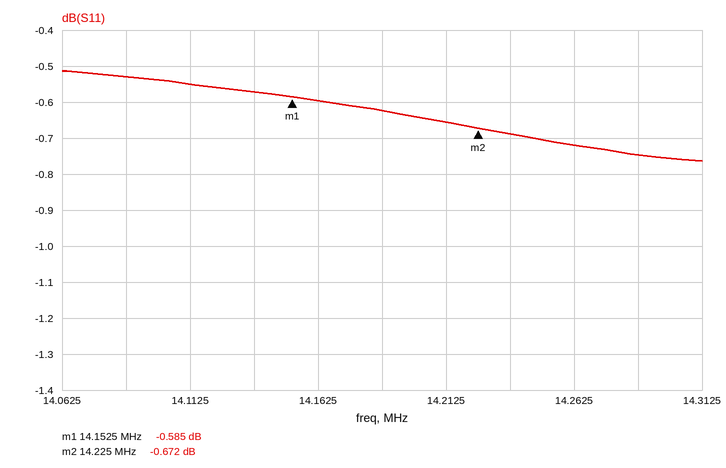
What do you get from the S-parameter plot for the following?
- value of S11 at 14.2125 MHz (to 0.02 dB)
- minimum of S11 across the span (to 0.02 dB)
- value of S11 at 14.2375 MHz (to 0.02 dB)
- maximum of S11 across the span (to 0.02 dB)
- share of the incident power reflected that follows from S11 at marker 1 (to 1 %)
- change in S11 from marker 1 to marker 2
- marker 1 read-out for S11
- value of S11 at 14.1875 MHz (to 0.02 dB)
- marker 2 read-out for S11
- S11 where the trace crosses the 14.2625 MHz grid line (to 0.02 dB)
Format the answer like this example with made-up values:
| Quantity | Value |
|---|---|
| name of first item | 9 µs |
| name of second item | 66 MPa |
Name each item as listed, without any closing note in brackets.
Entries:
| Quantity | Value |
|---|---|
| value of S11 at 14.2125 MHz | -0.66 dB |
| minimum of S11 across the span | -0.76 dB |
| value of S11 at 14.2375 MHz | -0.68 dB |
| maximum of S11 across the span | -0.52 dB |
| share of the incident power reflected that follows from S11 at marker 1 | 87 % |
| change in S11 from marker 1 to marker 2 | -0.087 dB |
| marker 1 read-out for S11 | -0.585 dB |
| value of S11 at 14.1875 MHz | -0.62 dB |
| marker 2 read-out for S11 | -0.672 dB |
| S11 where the trace crosses the 14.2625 MHz grid line | -0.72 dB |
